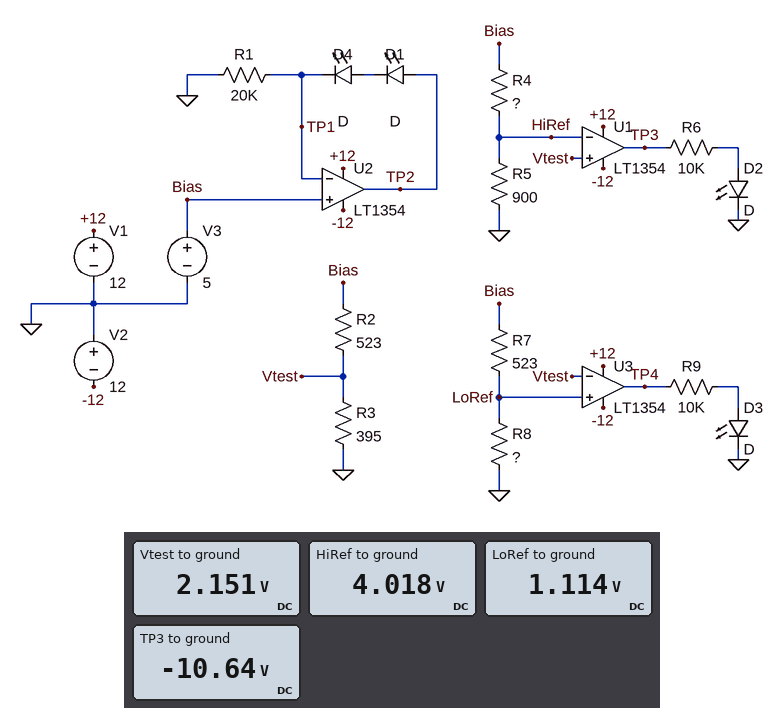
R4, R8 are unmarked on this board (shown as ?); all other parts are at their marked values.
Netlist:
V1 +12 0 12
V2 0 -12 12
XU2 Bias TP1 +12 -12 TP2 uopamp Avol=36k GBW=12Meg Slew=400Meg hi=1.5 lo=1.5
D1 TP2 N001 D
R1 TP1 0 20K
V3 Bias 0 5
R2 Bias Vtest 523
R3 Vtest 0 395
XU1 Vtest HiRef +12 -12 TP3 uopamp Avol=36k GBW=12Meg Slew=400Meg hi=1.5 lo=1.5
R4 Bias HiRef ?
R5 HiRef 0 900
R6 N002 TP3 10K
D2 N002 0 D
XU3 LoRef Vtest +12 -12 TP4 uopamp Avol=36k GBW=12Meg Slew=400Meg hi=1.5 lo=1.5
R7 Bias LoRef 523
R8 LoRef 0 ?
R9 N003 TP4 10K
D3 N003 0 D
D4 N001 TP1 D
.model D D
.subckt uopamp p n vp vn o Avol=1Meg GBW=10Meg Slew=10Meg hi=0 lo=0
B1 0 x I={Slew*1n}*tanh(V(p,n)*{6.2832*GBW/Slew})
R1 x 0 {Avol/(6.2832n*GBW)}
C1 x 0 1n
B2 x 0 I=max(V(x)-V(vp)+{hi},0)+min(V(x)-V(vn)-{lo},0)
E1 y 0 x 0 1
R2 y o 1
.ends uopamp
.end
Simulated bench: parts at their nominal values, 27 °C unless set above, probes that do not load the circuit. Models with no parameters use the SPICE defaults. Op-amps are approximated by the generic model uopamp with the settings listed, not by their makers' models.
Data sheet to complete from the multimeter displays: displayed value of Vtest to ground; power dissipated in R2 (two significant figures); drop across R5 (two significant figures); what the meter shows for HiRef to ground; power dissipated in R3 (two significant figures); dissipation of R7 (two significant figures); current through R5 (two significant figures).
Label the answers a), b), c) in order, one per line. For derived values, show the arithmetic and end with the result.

a) 2.151 V
b) (5 V - 2.151 V)^2 / 523 Ω = 16 mW
c) 4.018 V = 4.0 V
d) 4.018 V
e) (2.151 V)^2 / 395 Ω = 12 mW
f) (5 V - 1.114 V)^2 / 523 Ω = 29 mW
g) (4.018 V) / 900 Ω = 4.5 mA
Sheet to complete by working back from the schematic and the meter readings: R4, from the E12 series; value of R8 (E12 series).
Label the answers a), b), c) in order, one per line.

a) 220 Ω
b) 150 Ω
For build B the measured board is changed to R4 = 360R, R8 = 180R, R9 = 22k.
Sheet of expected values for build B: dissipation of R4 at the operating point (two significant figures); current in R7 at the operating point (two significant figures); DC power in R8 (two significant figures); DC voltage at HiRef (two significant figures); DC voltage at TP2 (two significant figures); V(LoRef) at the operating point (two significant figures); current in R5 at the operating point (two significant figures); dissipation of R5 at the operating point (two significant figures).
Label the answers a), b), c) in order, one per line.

a) 5.7 mW
b) 7.1 mA
c) 9.1 mW
d) 3.6 V
e) 6.2 V
f) 1.3 V
g) 4.0 mA
h) 14 mW
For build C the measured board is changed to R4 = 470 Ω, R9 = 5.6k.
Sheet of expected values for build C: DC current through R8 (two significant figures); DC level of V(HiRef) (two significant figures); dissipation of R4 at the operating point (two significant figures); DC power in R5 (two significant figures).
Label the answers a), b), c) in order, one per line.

a) 7.4 mA
b) 3.3 V
c) 6.3 mW
d) 12 mW
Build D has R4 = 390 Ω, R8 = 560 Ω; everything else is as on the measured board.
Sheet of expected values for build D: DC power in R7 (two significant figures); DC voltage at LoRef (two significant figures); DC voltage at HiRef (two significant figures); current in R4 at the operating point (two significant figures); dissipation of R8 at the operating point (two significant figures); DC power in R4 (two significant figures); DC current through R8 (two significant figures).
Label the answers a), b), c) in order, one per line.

a) 11 mW
b) 2.6 V
c) 3.5 V
d) 3.9 mA
e) 12 mW
f) 5.9 mW
g) 4.6 mA
